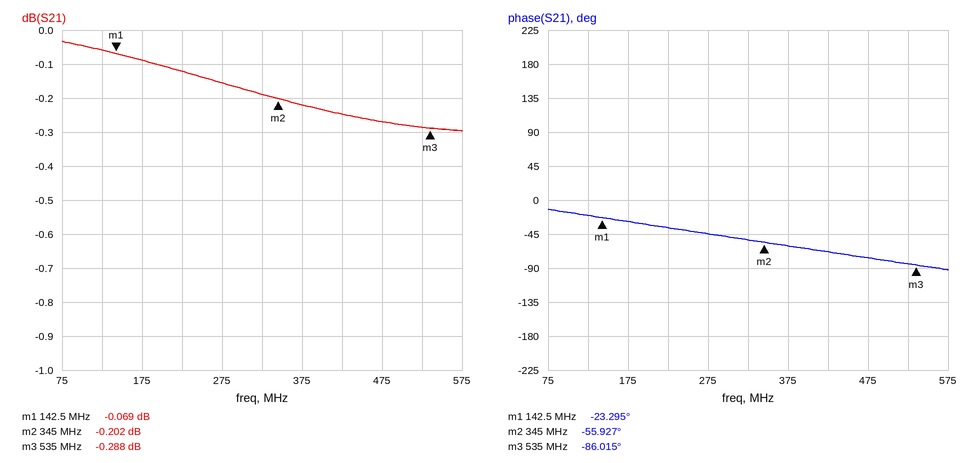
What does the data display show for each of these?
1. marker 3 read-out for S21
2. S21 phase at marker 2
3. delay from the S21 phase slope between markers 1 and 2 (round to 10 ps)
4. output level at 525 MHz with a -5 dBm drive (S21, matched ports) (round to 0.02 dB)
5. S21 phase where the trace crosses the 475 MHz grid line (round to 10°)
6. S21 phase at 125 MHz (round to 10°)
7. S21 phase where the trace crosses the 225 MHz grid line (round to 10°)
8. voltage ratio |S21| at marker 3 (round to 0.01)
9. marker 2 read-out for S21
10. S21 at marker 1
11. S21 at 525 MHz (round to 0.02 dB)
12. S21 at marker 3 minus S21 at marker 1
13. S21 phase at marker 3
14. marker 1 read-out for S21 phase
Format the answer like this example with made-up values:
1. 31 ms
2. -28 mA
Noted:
1. -0.288 dB
2. -55.927°
3. 450 ps
4. -5.28 dBm
5. -80°
6. -20°
7. -40°
8. 0.97
9. -0.202 dB
10. -0.069 dB
11. -0.28 dB
12. -0.219 dB
13. -86.015°
14. -23.295°
